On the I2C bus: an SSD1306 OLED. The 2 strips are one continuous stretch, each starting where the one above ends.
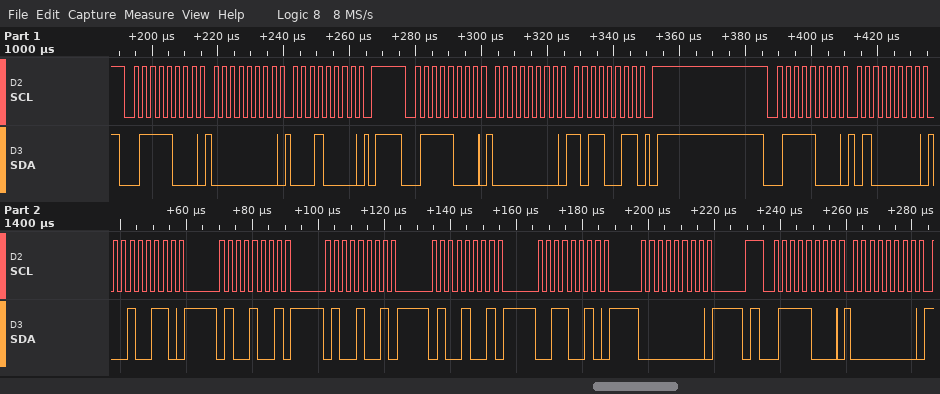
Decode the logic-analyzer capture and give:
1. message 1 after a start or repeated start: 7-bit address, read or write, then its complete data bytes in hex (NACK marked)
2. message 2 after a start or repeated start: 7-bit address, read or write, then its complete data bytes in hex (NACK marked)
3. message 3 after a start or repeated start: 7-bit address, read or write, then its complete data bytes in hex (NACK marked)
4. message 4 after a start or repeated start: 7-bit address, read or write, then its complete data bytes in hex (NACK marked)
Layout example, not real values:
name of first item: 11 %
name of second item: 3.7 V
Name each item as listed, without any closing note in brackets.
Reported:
message 1 after a start or repeated start: 7-bit address, read or write, then its complete data bytes in hex: 0x3C write: 00 10
message 2 after a start or repeated start: 7-bit address, read or write, then its complete data bytes in hex: 0x3C write: 00 B3
message 3 after a start or repeated start: 7-bit address, read or write, then its complete data bytes in hex: 0x3C write: 40 26 49 49 49 32 00
message 4 after a start or repeated start: 7-bit address, read or write, then its complete data bytes in hex: 0x3C write: 00
